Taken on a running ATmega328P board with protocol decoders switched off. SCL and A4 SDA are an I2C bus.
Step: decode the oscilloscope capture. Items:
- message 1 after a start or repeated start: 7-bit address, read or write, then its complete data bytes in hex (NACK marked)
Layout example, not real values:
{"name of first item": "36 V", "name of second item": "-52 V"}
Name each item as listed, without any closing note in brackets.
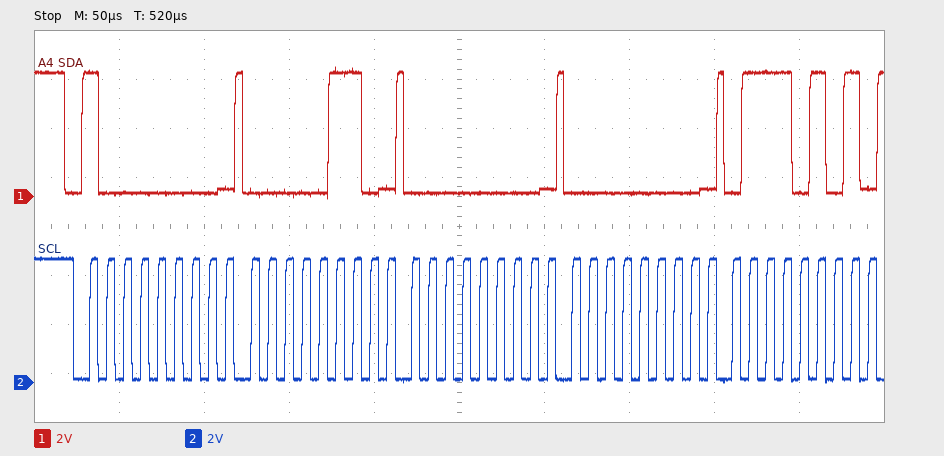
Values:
{"message 1 after a start or repeated start: 7-bit address, read or write, then its complete data bytes in hex": "0x40 write: 06 00 00 75"}
